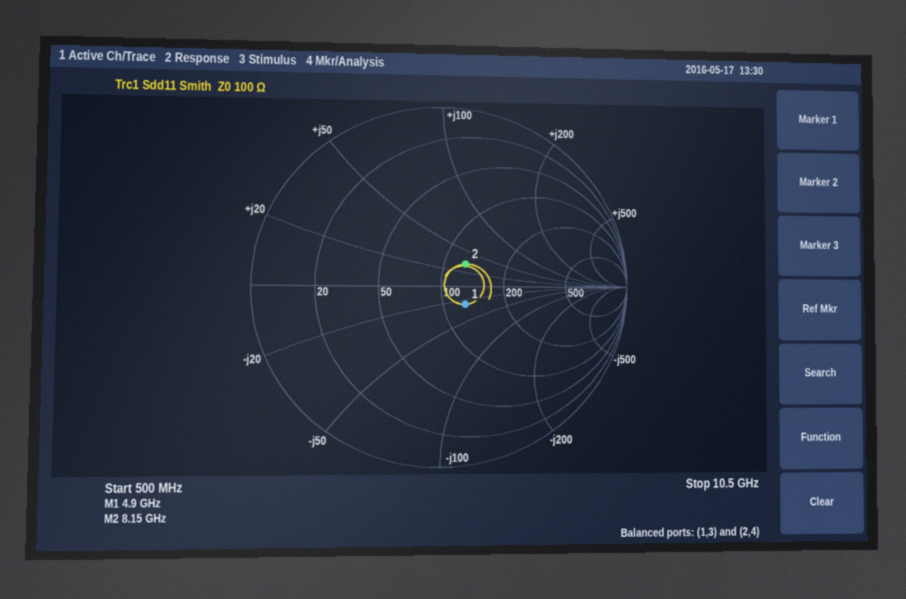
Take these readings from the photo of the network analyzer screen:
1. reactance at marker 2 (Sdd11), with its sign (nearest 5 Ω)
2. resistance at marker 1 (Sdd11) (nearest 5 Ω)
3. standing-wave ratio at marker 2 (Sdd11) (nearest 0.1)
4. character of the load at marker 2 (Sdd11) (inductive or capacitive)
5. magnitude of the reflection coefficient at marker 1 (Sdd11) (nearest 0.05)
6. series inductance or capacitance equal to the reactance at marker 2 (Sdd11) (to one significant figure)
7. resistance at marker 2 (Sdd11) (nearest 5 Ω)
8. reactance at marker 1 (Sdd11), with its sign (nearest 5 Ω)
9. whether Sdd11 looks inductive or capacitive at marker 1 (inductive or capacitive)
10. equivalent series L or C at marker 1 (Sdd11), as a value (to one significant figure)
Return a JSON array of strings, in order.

["+30 Ω", "125 Ω", "1.4", "inductive", "0.15", "600 pH", "125 Ω", "-25 Ω", "capacitive", "1 pF"]
